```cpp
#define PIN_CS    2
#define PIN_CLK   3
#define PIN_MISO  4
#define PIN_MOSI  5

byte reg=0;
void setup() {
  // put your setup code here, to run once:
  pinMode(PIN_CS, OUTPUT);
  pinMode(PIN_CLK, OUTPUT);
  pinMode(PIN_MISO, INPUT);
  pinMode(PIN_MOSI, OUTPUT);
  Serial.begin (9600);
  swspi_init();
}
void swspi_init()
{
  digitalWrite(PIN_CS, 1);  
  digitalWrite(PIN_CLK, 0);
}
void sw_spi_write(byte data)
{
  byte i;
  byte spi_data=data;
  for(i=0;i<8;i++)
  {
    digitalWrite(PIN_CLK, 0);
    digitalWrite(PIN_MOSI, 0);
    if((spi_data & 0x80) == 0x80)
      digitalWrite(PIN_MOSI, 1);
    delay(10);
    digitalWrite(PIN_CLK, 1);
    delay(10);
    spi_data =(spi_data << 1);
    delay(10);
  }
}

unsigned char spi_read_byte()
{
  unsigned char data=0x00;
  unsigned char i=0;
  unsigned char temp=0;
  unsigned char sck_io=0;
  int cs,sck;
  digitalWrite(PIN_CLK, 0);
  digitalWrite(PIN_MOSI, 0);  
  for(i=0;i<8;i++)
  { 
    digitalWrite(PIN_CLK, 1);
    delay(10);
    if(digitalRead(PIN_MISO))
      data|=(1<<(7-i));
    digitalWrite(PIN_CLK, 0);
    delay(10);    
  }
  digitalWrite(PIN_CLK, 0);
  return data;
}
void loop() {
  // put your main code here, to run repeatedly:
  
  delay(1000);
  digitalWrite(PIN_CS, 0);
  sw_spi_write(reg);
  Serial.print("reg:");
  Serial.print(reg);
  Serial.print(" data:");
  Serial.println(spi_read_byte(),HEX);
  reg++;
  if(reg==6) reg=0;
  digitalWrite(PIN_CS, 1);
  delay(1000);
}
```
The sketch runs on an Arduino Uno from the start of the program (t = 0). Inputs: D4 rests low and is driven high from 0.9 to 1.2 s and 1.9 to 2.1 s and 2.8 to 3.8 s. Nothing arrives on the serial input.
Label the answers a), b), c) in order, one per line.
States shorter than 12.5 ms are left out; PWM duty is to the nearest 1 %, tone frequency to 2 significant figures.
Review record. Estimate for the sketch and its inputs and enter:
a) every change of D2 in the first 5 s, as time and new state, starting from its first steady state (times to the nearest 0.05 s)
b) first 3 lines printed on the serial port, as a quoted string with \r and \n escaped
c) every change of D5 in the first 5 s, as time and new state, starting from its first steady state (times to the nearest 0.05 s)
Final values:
a) 0 s high; 1 s low; 1.4 s high; 3.4 s low; 3.8 s high
b) "reg:0 data:0\r\nreg:1 data:FF\r\nreg:2 data:0\r\n"
c) 0 s low; 3.6 s high; 3.65 s low
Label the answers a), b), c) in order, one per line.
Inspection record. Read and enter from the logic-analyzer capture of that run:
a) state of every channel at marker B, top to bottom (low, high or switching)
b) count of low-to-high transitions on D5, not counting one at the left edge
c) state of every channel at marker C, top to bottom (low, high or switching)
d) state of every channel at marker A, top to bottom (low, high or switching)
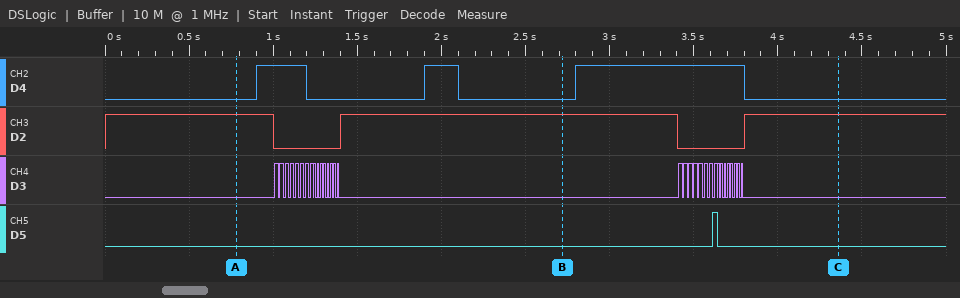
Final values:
a) D4 low, D2 high, D3 low, D5 low
b) 1
c) D4 low, D2 high, D3 low, D5 low
d) D4 low, D2 high, D3 low, D5 low
